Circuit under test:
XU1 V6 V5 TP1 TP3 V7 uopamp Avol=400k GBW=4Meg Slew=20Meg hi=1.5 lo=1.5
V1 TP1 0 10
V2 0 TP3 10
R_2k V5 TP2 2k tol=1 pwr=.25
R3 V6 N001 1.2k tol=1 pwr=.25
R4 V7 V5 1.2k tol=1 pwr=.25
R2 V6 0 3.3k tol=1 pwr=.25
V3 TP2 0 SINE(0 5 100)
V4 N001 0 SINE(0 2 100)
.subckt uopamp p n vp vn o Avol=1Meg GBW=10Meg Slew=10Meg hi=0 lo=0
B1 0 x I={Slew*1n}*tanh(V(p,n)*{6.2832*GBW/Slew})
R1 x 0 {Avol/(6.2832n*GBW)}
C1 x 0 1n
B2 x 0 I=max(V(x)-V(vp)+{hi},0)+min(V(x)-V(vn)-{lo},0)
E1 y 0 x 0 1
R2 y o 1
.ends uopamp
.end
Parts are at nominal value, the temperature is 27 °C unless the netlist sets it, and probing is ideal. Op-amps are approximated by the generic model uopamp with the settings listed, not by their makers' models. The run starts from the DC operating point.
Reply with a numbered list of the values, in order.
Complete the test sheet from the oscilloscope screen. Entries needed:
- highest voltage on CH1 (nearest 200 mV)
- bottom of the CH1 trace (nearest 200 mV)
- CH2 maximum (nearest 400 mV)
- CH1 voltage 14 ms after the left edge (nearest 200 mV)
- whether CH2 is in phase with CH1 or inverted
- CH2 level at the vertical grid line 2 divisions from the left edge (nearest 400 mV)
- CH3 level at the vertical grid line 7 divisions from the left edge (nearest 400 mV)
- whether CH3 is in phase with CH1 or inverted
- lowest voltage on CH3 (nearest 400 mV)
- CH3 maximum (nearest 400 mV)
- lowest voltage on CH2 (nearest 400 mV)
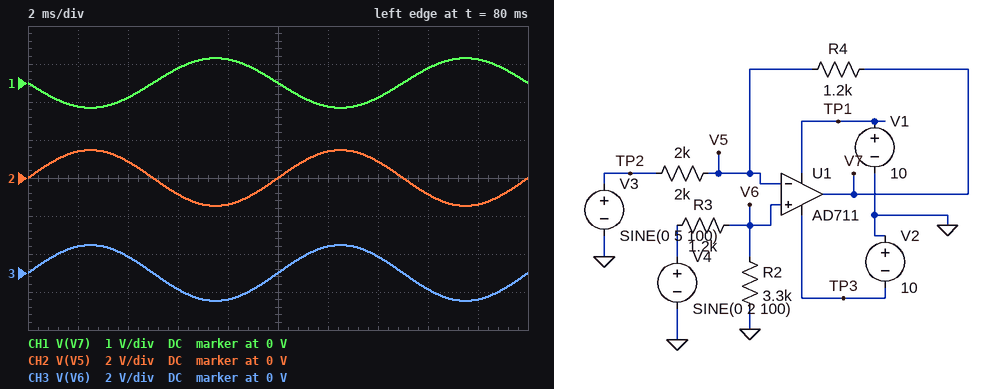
1. 600 mV
2. -600 mV
3. 1.6 V
4. -400 mV
5. inverted
6. 800 mV
7. 800 mV
8. inverted
9. -1.6 V
10. 1.6 V
11. -1.6 V
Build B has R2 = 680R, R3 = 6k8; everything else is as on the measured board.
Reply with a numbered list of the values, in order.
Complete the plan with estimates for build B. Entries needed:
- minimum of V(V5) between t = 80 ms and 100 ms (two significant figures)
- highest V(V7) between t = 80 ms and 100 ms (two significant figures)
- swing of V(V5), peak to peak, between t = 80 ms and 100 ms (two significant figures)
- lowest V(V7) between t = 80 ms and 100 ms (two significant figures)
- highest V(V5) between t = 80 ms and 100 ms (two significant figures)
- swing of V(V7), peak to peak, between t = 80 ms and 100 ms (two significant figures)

1. -180 mV
2. 2.7 V
3. 360 mV
4. -2.7 V
5. 180 mV
6. 5.4 V
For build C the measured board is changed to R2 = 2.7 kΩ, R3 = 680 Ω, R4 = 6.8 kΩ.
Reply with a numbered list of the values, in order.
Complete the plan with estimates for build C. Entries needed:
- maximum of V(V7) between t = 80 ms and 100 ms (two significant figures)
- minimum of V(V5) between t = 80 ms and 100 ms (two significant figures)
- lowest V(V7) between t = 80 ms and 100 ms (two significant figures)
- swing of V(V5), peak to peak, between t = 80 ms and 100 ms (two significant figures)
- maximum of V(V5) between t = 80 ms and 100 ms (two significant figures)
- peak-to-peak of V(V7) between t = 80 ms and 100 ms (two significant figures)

1. 8.5 V
2. -1.9 V
3. -8.5 V
4. 3.9 V
5. 1.9 V
6. 17 V
